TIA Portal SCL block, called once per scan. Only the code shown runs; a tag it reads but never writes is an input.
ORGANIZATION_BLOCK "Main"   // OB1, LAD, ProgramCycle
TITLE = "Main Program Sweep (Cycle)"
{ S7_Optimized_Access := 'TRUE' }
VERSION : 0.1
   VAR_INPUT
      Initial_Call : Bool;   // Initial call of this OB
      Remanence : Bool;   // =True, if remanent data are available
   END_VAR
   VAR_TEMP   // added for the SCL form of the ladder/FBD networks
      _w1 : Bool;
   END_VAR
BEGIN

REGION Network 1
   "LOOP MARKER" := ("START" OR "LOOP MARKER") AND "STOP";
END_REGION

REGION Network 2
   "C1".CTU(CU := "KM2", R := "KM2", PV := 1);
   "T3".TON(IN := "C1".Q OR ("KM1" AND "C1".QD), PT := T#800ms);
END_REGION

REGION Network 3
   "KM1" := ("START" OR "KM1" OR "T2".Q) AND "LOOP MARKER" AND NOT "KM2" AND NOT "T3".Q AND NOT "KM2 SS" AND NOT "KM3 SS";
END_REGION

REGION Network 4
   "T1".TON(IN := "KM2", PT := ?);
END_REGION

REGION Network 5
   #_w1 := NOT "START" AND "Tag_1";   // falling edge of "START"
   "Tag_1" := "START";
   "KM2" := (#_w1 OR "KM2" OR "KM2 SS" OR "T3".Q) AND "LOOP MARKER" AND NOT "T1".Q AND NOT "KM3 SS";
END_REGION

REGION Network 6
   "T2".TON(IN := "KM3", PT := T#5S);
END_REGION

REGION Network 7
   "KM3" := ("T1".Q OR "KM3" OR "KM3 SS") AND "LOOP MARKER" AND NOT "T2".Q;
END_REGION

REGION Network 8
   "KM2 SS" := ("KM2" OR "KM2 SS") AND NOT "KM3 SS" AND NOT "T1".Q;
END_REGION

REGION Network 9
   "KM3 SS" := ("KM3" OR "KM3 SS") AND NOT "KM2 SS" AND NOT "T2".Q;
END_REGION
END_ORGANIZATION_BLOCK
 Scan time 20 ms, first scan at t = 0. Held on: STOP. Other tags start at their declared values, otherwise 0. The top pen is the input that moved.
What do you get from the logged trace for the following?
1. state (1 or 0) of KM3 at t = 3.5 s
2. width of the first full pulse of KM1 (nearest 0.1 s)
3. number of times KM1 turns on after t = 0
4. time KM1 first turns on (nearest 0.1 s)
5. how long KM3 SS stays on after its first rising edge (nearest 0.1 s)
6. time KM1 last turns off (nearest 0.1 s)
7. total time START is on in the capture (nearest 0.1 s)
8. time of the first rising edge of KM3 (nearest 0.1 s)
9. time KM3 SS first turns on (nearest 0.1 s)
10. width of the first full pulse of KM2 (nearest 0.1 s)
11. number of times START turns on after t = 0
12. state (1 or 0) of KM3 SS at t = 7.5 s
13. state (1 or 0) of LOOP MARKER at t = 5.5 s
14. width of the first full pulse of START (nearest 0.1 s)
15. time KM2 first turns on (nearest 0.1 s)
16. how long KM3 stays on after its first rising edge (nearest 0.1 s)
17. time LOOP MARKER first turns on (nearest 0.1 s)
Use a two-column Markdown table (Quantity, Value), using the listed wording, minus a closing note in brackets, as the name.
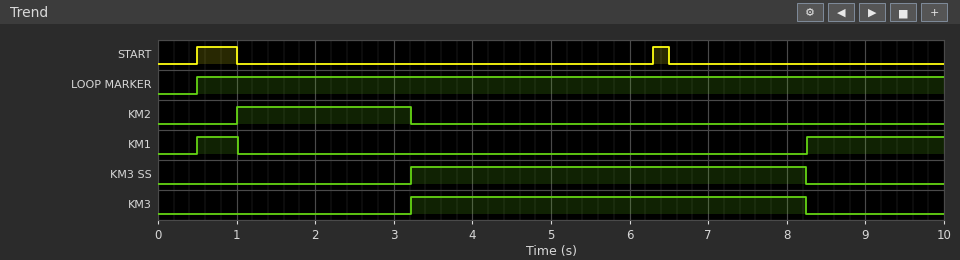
| Quantity | Value |
|---|---|
| state (1 or 0) of KM3 at t = 3.5 s | 1 |
| width of the first full pulse of KM1 | 0.5 s |
| number of times KM1 turns on after t = 0 | 2 |
| time KM1 first turns on | 0.5 s |
| how long KM3 SS stays on after its first rising edge | 5.0 s |
| time KM1 last turns off | 1.0 s |
| total time START is on in the capture | 0.7 s |
| time of the first rising edge of KM3 | 3.2 s |
| time KM3 SS first turns on | 3.2 s |
| width of the first full pulse of KM2 | 2.2 s |
| number of times START turns on after t = 0 | 2 |
| state (1 or 0) of KM3 SS at t = 7.5 s | 1 |
| state (1 or 0) of LOOP MARKER at t = 5.5 s | 1 |
| width of the first full pulse of START | 0.5 s |
| time KM2 first turns on | 1.0 s |
| how long KM3 stays on after its first rising edge | 5.0 s |
| time LOOP MARKER first turns on | 0.5 s |
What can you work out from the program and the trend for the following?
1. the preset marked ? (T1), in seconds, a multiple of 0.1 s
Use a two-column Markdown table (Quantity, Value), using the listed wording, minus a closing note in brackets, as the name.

| Quantity | Value |
|---|---|
| the preset marked ? (T1), in seconds, a multiple of 0.1 s | 2.2 s |
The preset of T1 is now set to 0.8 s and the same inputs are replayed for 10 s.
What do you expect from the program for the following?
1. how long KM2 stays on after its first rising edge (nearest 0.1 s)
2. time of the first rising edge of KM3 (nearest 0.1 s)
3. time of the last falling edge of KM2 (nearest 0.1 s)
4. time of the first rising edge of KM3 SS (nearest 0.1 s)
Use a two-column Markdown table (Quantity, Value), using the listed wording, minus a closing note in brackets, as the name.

| Quantity | Value |
|---|---|
| how long KM2 stays on after its first rising edge | 0.8 s |
| time of the first rising edge of KM3 | 1.8 s |
| time of the last falling edge of KM2 | 1.8 s |
| time of the first rising edge of KM3 SS | 1.8 s |
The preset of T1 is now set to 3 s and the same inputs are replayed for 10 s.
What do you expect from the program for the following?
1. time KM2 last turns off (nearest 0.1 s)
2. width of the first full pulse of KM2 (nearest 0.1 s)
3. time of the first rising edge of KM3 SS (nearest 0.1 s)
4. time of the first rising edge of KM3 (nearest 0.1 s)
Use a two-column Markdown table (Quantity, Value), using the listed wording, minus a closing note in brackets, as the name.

| Quantity | Value |
|---|---|
| time KM2 last turns off | 4.0 s |
| width of the first full pulse of KM2 | 3.0 s |
| time of the first rising edge of KM3 SS | 4.0 s |
| time of the first rising edge of KM3 | 4.0 s |
